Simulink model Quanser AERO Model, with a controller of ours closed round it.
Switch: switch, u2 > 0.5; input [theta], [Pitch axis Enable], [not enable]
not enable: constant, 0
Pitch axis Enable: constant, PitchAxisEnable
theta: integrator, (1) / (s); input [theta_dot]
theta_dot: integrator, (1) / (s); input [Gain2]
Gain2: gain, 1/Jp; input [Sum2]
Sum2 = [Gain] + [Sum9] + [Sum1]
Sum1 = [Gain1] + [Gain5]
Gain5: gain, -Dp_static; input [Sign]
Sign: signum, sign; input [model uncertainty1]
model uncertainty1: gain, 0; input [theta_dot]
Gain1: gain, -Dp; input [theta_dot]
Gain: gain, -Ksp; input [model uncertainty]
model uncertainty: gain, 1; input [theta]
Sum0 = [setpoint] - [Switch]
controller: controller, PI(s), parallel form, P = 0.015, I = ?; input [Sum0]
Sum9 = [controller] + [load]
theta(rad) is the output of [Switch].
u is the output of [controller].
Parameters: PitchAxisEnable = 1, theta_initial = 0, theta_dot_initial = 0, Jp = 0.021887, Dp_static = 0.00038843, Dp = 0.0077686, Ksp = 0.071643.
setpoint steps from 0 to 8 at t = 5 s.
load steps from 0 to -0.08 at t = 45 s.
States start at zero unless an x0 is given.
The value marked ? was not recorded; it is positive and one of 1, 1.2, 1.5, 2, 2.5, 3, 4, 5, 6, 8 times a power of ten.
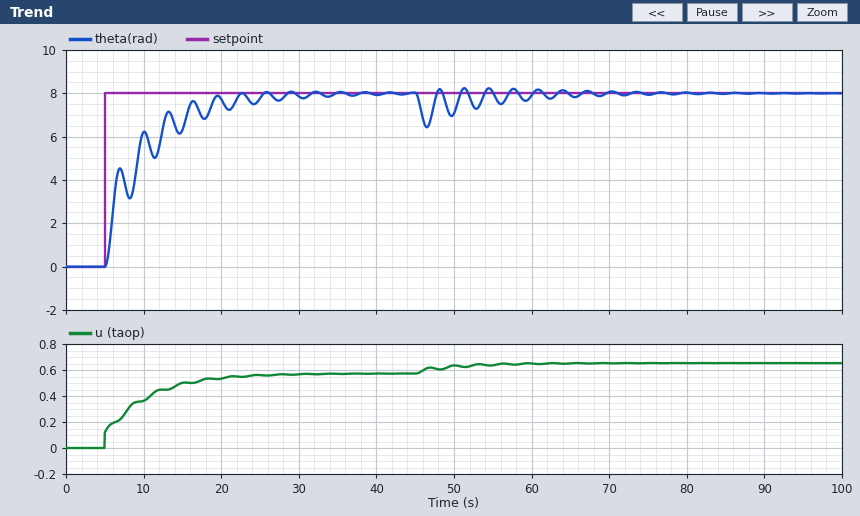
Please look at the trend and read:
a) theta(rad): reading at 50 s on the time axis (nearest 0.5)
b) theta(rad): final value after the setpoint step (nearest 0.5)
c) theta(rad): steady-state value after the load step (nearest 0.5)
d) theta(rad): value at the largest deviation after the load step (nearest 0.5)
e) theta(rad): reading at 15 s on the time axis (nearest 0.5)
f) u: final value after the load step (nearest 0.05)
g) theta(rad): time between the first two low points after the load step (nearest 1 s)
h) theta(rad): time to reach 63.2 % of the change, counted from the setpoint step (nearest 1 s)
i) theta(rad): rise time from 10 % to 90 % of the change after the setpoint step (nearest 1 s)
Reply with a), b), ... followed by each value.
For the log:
a) 7.0
b) 8.0
c) 8.0
d) 6.5
e) 6.5
f) 0.65
g) 3 s
h) 4 s
i) 10 s
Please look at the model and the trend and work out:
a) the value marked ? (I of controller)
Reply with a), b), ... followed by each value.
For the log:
a) 0.015
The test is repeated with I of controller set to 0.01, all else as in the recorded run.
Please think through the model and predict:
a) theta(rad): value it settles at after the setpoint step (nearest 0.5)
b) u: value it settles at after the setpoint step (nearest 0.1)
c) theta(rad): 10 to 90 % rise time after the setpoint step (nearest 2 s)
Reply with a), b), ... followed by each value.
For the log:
a) 8.0
b) 0.6
c) 16 s
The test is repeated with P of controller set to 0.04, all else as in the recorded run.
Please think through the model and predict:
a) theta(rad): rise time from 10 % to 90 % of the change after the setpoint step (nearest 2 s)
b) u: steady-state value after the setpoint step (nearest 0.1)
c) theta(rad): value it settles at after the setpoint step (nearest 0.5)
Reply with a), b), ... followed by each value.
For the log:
a) 6 s
b) 0.6
c) 8.0
